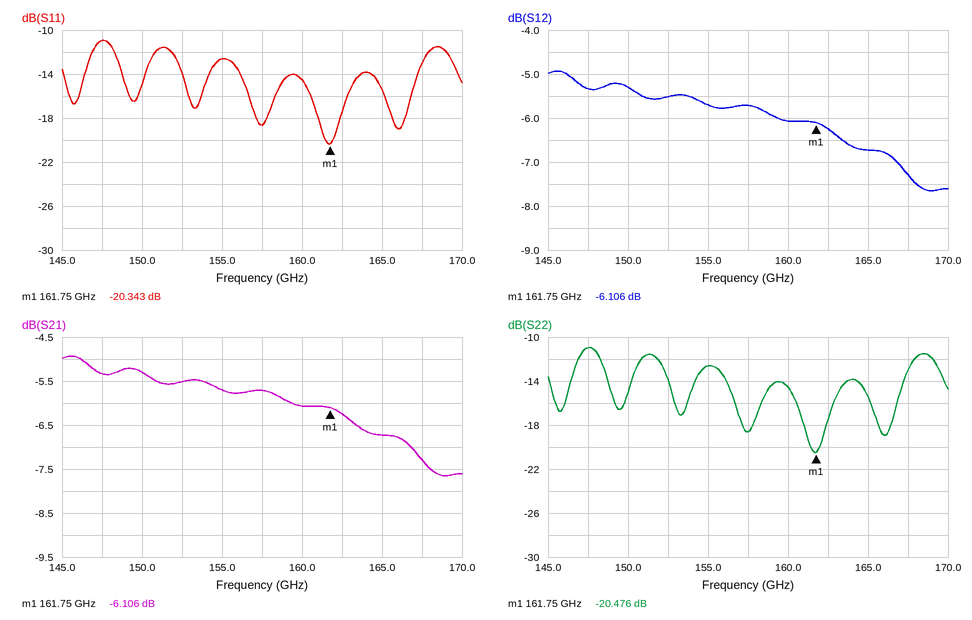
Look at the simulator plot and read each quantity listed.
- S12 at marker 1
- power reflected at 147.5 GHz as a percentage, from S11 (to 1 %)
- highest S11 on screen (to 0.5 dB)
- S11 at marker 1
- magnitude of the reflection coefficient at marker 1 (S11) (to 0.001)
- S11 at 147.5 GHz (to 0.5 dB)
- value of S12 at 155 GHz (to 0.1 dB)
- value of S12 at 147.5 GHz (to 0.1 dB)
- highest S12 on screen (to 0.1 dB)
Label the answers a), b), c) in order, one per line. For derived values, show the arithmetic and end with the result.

a) -6.106 dB
b) 10^(-11/10) ≈ 8 %
c) -11.0 dB
d) -20.343 dB
e) 10^(-20.343/20) ≈ 0.096
f) -11.0 dB
g) -5.7 dB
h) -5.3 dB
i) -4.9 dB
